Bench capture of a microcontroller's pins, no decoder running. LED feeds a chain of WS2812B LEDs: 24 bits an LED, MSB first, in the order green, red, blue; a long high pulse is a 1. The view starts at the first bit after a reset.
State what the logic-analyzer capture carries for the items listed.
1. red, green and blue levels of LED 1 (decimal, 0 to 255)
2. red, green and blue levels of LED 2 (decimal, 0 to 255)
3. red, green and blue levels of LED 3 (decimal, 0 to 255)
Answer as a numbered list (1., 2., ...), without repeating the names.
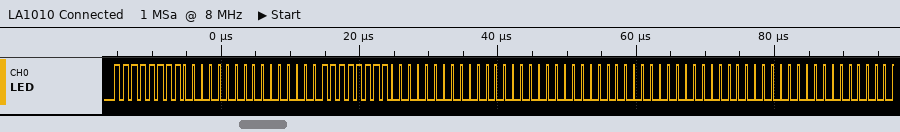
1. 0, 255, 0
2. 0, 255, 0
3. 0, 0, 0
